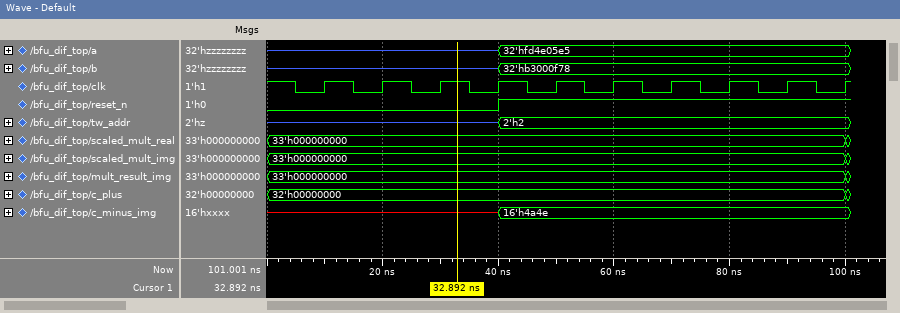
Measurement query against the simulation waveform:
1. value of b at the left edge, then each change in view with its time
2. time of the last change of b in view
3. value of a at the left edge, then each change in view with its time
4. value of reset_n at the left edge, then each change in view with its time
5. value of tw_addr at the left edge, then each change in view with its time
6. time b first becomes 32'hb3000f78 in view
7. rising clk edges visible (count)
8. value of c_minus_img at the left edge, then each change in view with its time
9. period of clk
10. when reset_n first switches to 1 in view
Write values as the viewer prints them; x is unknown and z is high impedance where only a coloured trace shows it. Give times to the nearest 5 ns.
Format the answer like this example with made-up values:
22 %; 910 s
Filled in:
z, 32'hb3000f78 at 40 ns; 40 ns; z, 32'hfd4e05e5 at 40 ns; 0, 1 at 40 ns; z, 2'h2 at 40 ns; 40 ns; 10; x, 16'h4a4e at 40 ns; 10 ns; 40 ns
